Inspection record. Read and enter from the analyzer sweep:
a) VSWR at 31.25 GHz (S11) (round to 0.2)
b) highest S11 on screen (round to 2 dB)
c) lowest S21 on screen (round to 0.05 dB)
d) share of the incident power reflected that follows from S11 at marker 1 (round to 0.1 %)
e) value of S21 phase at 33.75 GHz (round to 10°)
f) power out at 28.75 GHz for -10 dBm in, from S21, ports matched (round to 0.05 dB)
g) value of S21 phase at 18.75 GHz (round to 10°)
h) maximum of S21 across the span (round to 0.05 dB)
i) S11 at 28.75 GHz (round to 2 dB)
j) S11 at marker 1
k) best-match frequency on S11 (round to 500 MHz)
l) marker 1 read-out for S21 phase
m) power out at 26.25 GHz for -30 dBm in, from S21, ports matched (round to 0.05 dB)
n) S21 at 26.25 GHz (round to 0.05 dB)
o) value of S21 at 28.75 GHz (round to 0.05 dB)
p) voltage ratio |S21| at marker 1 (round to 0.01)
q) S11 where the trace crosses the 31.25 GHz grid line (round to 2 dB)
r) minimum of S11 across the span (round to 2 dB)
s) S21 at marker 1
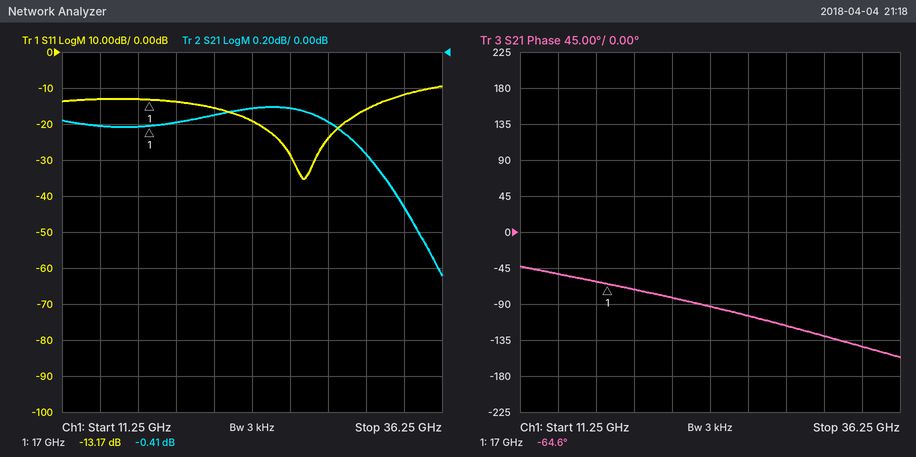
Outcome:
1.4
-10 dB
-1.25 dB
4.8 %
-140°
-10.40 dBm
-70°
-0.30 dB
-24 dB
-13.17 dB
27.0 GHz
-64.6°
-30.30 dBm
-0.30 dB
-0.40 dB
0.95
-16 dB
-36 dB
-0.41 dB
